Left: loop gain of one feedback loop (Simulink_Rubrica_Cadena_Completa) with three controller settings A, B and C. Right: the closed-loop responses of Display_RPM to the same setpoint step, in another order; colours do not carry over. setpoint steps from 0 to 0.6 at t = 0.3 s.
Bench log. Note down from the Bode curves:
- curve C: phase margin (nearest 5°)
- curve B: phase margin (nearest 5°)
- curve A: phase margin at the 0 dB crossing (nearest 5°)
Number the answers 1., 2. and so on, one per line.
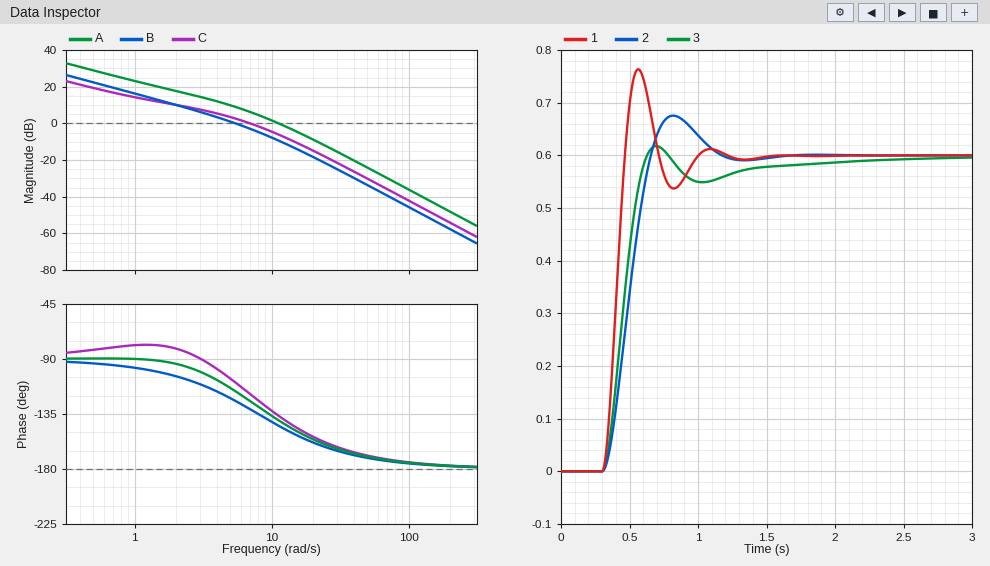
1. 60°
2. 55°
3. 40°
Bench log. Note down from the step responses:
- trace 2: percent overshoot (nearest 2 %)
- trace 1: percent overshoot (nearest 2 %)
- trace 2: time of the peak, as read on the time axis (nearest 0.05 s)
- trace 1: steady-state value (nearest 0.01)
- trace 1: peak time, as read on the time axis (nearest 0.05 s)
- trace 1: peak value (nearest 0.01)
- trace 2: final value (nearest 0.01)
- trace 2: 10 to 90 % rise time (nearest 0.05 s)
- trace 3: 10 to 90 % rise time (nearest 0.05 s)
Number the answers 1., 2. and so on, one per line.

1. 12 %
2. 28 %
3. 0.80 s
4. 0.60
5. 0.55 s
6. 0.76
7. 0.60
8. 0.25 s
9. 0.20 s
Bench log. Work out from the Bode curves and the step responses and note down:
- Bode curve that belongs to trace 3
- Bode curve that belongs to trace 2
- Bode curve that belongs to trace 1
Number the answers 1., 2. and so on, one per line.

1. C
2. B
3. A
